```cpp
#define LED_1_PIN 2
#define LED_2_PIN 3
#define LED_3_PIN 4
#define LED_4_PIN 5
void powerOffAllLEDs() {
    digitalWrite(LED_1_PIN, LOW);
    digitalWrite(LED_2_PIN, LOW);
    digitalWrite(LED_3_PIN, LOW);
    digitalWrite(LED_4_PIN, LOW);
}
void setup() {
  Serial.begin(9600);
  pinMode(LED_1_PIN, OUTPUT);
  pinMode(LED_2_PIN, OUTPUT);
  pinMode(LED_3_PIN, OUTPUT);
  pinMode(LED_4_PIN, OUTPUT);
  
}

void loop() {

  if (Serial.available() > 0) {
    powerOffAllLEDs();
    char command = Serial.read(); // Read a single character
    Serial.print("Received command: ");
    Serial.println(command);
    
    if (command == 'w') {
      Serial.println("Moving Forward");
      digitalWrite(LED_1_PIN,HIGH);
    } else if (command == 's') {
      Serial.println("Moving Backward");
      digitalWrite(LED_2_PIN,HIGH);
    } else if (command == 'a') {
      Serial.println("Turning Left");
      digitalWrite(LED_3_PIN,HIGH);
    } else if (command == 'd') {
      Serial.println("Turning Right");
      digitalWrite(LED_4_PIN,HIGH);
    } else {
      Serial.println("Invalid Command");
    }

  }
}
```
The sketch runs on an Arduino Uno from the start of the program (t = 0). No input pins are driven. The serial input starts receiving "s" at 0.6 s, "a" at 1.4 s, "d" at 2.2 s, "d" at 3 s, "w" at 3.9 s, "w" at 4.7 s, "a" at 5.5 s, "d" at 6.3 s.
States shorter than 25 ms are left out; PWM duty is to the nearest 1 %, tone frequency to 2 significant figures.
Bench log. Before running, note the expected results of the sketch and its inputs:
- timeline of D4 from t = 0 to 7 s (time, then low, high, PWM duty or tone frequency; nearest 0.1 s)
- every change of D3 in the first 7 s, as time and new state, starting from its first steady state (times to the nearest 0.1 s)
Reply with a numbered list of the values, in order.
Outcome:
1. 0 s low; 1.4 s high; 2.2 s low; 5.5 s high; 6.3 s low
2. 0 s low; 0.6 s high; 1.4 s low
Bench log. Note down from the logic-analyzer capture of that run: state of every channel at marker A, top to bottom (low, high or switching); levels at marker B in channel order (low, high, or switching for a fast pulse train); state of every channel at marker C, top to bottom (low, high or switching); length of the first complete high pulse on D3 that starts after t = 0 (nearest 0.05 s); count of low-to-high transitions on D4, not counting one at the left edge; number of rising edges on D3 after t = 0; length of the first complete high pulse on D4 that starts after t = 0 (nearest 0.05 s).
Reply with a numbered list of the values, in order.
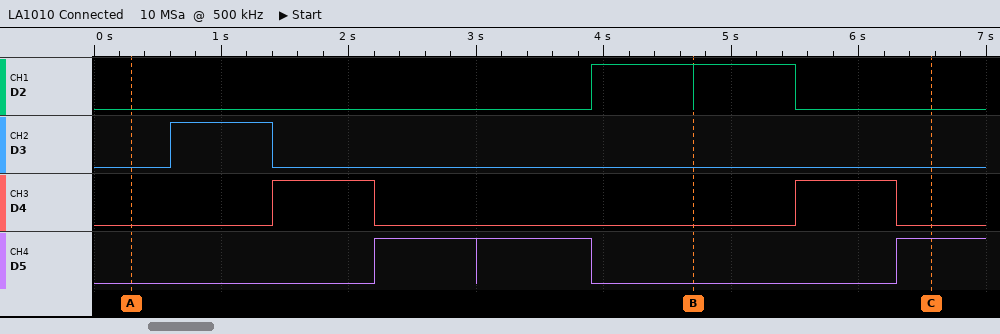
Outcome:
1. D2 low, D3 low, D4 low, D5 low
2. D2 high, D3 low, D4 low, D5 low
3. D2 low, D3 low, D4 low, D5 high
4. 0.80 s
5. 2
6. 1
7. 0.80 s
